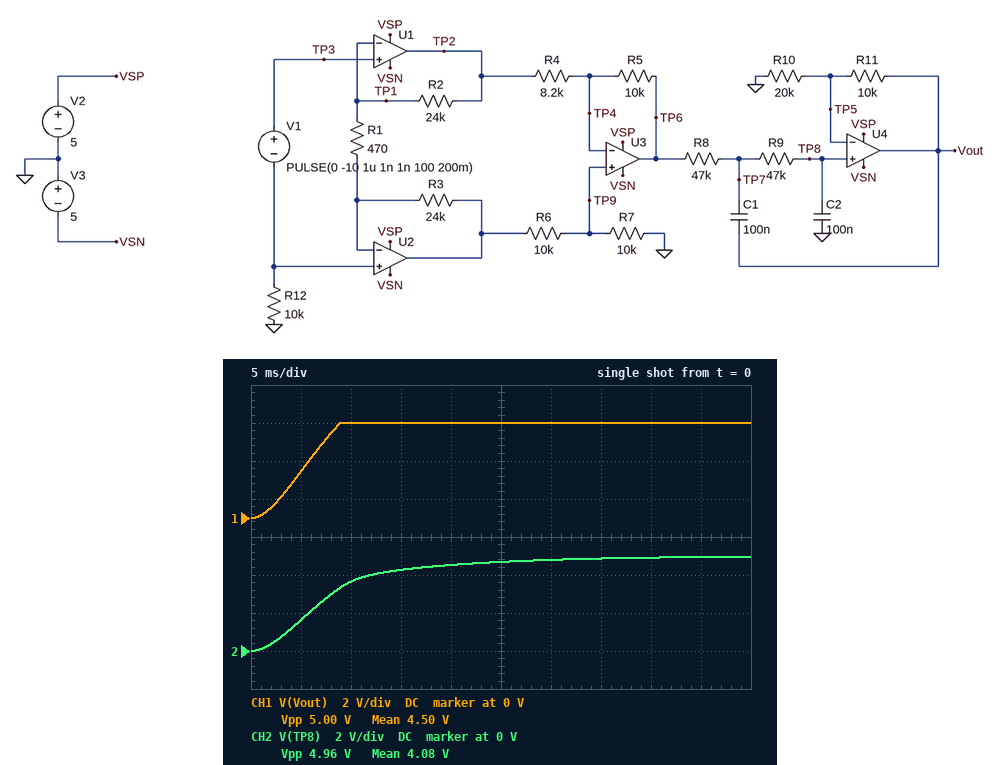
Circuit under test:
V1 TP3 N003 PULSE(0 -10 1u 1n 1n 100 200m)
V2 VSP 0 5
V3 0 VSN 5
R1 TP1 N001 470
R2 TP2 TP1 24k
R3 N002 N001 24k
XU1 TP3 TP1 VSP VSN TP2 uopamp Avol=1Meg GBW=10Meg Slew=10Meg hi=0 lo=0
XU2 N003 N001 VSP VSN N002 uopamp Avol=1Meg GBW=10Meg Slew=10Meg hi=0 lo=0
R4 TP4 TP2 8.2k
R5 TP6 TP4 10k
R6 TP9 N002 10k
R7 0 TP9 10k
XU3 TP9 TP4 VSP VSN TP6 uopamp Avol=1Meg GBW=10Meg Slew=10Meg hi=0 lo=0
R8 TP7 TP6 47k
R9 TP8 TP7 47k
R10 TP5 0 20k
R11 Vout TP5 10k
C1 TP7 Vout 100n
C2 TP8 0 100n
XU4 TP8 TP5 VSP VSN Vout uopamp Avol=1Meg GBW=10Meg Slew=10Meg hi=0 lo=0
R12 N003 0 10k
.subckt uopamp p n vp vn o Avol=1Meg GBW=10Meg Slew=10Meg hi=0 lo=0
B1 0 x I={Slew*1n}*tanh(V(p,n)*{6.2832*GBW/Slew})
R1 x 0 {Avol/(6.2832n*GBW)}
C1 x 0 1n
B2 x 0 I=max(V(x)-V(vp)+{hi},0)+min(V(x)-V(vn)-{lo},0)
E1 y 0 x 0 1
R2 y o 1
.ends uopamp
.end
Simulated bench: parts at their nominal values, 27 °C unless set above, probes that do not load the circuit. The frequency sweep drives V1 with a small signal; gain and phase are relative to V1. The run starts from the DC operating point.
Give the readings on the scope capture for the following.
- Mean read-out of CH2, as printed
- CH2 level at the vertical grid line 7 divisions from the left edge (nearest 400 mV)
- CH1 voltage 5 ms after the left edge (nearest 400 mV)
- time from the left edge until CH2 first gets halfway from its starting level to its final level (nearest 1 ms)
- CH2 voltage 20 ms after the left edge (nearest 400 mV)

4.08 V
4.8 V
2.4 V
7 ms
4.4 V
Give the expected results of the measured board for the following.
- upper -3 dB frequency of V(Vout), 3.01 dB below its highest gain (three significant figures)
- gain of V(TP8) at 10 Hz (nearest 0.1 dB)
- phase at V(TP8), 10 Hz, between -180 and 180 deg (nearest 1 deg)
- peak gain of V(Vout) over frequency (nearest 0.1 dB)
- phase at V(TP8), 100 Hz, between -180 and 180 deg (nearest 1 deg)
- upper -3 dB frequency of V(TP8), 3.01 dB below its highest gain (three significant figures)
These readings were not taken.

31.8 Hz
41.5 dB
154 deg
45.1 dB
30 deg
31.8 Hz
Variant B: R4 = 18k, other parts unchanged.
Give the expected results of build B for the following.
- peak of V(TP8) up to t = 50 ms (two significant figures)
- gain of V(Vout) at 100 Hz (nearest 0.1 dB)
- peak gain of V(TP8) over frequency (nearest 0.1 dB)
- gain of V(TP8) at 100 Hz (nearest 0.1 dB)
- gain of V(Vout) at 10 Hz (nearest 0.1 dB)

5.0 V
21.3 dB
36.7 dB
17.7 dB
40.1 dB
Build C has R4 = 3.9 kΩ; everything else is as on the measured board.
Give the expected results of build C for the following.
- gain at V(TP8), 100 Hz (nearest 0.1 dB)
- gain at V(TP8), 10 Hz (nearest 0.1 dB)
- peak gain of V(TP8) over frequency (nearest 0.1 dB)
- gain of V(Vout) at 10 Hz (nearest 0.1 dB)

28.0 dB
46.9 dB
47.0 dB
50.4 dB
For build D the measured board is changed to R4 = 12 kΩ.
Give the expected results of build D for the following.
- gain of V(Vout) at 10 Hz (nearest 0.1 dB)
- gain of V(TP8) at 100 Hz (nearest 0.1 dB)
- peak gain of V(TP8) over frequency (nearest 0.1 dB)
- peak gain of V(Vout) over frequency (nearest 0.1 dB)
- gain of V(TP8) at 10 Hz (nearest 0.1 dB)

42.5 dB
20.1 dB
39.1 dB
42.6 dB
39.0 dB
